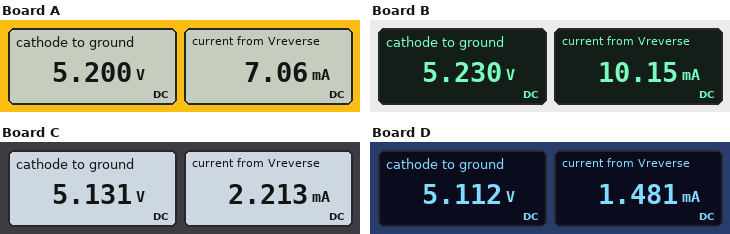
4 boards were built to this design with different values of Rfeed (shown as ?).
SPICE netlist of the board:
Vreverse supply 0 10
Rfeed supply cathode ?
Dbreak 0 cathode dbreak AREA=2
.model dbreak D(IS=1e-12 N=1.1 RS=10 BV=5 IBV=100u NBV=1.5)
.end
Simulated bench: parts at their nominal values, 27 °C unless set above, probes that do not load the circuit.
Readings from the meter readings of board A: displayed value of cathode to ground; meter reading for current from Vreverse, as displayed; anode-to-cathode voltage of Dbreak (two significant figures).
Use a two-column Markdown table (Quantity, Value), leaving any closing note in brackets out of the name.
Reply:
| Quantity | Value |
|---|---|
| displayed value of cathode to ground | 5.200 V |
| meter reading for current from Vreverse, as displayed | 7.06 mA |
| anode-to-cathode voltage of Dbreak | -5.2 V |
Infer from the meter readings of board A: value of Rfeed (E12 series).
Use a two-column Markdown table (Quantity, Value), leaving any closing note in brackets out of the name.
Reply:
| Quantity | Value |
|---|---|
| value of Rfeed | 680 Ω |
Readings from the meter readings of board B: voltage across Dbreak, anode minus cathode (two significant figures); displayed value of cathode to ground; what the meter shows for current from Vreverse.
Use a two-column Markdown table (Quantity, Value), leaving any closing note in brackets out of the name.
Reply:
| Quantity | Value |
|---|---|
| voltage across Dbreak, anode minus cathode | -5.2 V |
| displayed value of cathode to ground | 5.230 V |
| what the meter shows for current from Vreverse | 10.15 mA |
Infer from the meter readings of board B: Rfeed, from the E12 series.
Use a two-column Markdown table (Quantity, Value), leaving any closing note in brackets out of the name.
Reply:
| Quantity | Value |
|---|---|
| Rfeed, from the E12 series | 470 Ω |
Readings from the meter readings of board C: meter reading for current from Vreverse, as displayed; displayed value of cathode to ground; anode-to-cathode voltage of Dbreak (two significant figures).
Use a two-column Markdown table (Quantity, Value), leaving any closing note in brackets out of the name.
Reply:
| Quantity | Value |
|---|---|
| meter reading for current from Vreverse, as displayed | 2.213 mA |
| displayed value of cathode to ground | 5.131 V |
| anode-to-cathode voltage of Dbreak | -5.1 V |
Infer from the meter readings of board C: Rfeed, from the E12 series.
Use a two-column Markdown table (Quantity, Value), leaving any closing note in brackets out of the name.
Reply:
| Quantity | Value |
|---|---|
| Rfeed, from the E12 series | 2.2 kΩ |
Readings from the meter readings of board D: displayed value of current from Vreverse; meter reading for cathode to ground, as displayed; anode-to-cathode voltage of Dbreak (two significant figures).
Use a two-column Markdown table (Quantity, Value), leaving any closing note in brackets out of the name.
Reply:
| Quantity | Value |
|---|---|
| displayed value of current from Vreverse | 1.481 mA |
| meter reading for cathode to ground, as displayed | 5.112 V |
| anode-to-cathode voltage of Dbreak | -5.1 V |
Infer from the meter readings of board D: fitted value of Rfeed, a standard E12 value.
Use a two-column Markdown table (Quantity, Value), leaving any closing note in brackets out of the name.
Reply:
| Quantity | Value |
|---|---|
| fitted value of Rfeed, a standard E12 value | 3.3 kΩ |
